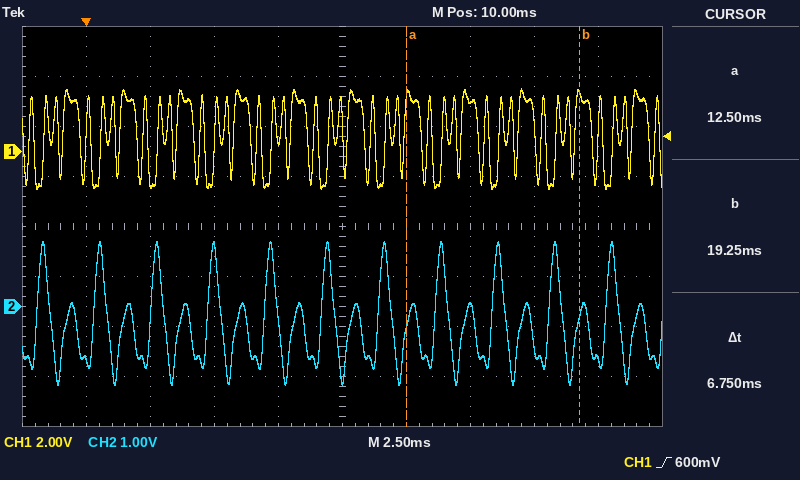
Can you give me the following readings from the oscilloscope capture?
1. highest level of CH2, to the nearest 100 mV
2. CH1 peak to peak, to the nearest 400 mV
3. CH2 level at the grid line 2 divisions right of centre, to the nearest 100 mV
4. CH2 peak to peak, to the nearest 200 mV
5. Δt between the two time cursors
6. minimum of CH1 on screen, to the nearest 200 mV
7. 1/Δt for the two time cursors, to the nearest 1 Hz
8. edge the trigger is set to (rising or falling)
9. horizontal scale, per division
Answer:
1.3 V
4.0 V
0.0 V
2.8 V
6.75 ms
-1.4 V
148 Hz
rising
2.5 ms
